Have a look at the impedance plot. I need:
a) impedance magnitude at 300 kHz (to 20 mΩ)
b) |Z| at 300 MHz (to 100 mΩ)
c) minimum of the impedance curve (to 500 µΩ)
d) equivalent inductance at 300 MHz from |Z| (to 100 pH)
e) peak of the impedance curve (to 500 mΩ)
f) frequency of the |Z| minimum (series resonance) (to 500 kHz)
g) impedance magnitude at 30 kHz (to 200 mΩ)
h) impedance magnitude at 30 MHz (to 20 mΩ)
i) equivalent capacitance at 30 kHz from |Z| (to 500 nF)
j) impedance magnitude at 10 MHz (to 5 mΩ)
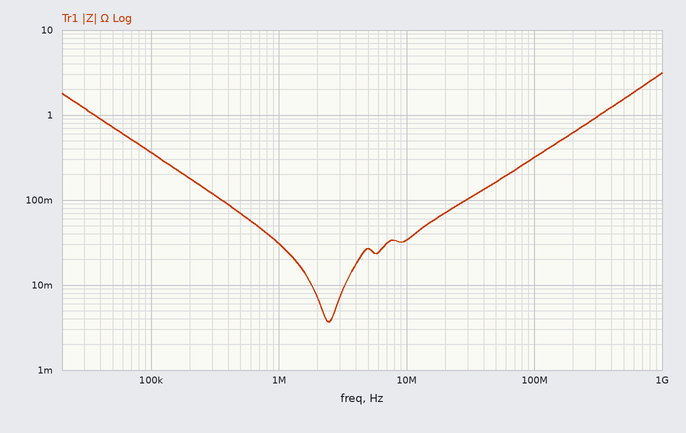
120 mΩ
900 mΩ
3.5 mΩ
500 pH
3.0 Ω
2.5 MHz
1.2 Ω
100 mΩ
4.5 µF
35 mΩ
